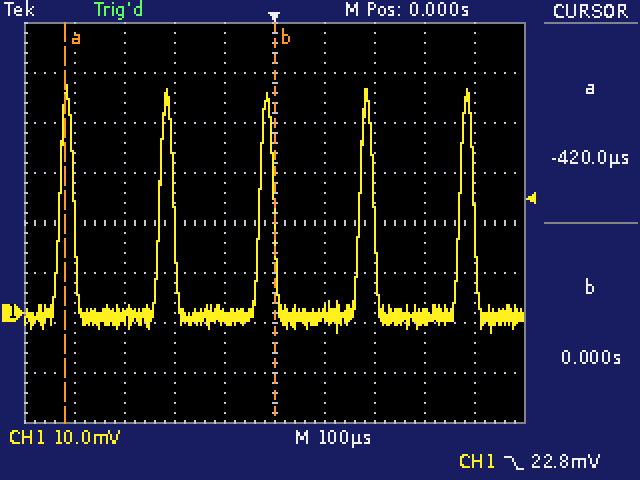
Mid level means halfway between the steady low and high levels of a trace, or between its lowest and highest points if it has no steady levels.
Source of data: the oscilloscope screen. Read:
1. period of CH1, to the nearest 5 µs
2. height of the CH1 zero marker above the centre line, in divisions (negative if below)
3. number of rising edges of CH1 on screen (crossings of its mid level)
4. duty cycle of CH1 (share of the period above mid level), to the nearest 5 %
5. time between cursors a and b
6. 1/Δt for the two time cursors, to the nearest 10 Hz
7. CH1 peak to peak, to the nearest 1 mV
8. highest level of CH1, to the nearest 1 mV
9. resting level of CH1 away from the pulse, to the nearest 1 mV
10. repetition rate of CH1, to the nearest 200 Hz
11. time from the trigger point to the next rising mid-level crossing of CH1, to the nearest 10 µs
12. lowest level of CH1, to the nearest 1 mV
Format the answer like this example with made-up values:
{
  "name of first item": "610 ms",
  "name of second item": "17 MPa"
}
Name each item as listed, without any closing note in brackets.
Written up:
{
  "period of CH1, to the nearest 5 µs": "200 µs",
  "height of the CH1 zero marker above the centre line, in divisions": "-1.8 div",
  "number of rising edges of CH1 on screen": "5",
  "duty cycle of CH1 (share of the period above mid level), to the nearest 5 %": "15 %",
  "time between cursors a and b": "420 µs",
  "1/Δt for the two time cursors, to the nearest 10 Hz": "2.38 kHz",
  "CH1 peak to peak, to the nearest 1 mV": "50 mV",
  "highest level of CH1, to the nearest 1 mV": "46 mV",
  "resting level of CH1 away from the pulse, to the nearest 1 mV": "-1 mV",
  "repetition rate of CH1, to the nearest 200 Hz": "5.0 kHz",
  "time from the trigger point to the next rising mid-level crossing of CH1, to the nearest 10 µs": "170 µs",
  "lowest level of CH1, to the nearest 1 mV": "-4 mV"
}
